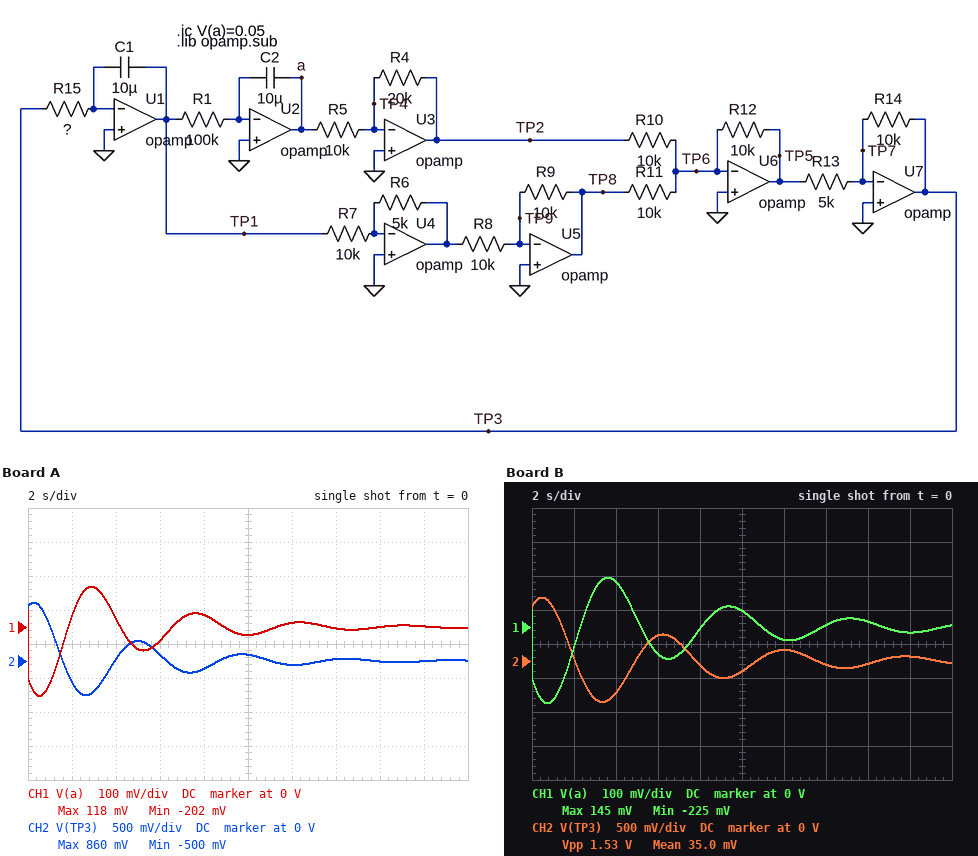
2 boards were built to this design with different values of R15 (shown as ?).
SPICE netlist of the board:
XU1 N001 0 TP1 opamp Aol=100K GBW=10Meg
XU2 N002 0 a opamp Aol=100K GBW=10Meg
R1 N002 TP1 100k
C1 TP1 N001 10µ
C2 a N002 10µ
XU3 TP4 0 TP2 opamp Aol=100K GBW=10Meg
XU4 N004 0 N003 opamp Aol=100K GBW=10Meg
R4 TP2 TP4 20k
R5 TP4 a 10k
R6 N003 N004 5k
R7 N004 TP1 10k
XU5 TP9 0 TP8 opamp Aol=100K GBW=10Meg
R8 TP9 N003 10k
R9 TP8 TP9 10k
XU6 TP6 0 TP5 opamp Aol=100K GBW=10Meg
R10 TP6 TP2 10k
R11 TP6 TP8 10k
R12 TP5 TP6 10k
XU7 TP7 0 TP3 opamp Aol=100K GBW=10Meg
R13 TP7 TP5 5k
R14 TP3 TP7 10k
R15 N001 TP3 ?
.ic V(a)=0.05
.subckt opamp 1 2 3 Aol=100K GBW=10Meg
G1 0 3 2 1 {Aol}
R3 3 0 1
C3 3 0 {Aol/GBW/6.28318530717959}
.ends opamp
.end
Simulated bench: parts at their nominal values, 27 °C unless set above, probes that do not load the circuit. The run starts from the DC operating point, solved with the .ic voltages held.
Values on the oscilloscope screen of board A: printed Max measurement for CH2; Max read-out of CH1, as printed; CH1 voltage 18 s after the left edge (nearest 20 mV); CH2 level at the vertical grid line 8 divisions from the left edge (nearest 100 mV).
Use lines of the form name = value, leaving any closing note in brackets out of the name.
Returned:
printed Max measurement for CH2 = 860 mV
Max read-out of CH1, as printed = 118 mV
CH1 voltage 18 s after the left edge = 0 V
CH2 level at the vertical grid line 8 divisions from the left edge = 0 V
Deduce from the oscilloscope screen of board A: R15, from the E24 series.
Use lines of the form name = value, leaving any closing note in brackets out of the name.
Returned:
R15, from the E24 series = 220 kΩ
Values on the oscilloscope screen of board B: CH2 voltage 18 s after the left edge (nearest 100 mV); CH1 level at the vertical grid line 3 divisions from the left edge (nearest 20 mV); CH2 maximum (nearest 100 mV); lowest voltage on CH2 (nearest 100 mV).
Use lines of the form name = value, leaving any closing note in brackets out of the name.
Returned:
CH2 voltage 18 s after the left edge = 100 mV
CH1 level at the vertical grid line 3 divisions from the left edge = -80 mV
CH2 maximum = 900 mV
lowest voltage on CH2 = -600 mV
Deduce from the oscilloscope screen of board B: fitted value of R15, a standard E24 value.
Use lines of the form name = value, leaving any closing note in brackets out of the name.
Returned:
fitted value of R15, a standard E24 value = 330 kΩ
